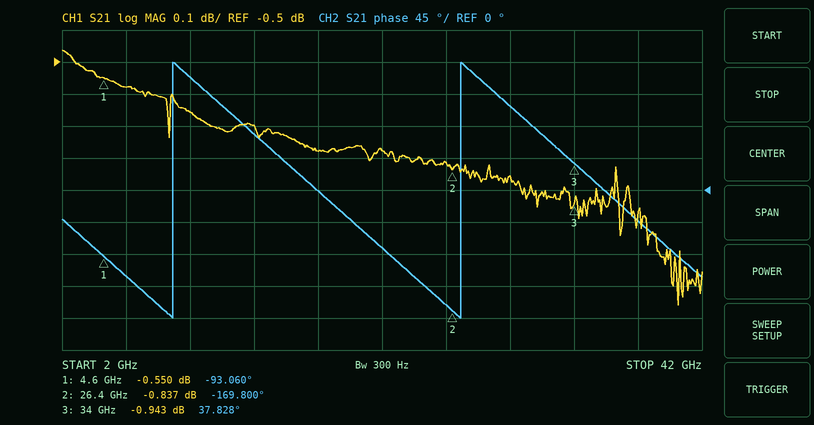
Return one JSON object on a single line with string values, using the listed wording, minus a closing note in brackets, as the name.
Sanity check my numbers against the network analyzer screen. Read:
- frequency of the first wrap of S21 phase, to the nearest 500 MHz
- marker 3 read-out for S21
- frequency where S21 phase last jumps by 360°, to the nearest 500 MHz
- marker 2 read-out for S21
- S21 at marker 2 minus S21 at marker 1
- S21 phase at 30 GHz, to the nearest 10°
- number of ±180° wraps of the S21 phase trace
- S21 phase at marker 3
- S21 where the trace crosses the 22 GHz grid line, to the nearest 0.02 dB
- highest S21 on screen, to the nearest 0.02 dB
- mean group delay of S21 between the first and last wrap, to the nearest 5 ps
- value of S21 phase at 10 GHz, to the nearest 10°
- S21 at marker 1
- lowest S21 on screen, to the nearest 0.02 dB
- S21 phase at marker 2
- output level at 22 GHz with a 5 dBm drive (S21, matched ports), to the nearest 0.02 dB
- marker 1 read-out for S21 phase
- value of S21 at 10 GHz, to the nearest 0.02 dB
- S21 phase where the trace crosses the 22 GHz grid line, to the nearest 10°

{"frequency of the first wrap of S21 phase, to the nearest 500 MHz": "9.0 GHz", "marker 3 read-out for S21": "-0.943 dB", "frequency where S21 phase last jumps by 360°, to the nearest 500 MHz": "27.0 GHz", "marker 2 read-out for S21": "-0.837 dB", "S21 at marker 2 minus S21 at marker 1": "-0.287 dB", "S21 phase at 30 GHz, to the nearest 10°": "120°", "number of ±180° wraps of the S21 phase trace": "2", "S21 phase at marker 3": "37.828°", "S21 where the trace crosses the 22 GHz grid line, to the nearest 0.02 dB": "-0.78 dB", "highest S21 on screen, to the nearest 0.02 dB": "-0.46 dB", "mean group delay of S21 between the first and last wrap, to the nearest 5 ps": "55 ps", "value of S21 phase at 10 GHz, to the nearest 10°": "160°", "S21 at marker 1": "-0.550 dB", "lowest S21 on screen, to the nearest 0.02 dB": "-1.26 dB", "S21 phase at marker 2": "-169.800°", "output level at 22 GHz with a 5 dBm drive (S21, matched ports), to the nearest 0.02 dB": "4.22 dBm", "marker 1 read-out for S21 phase": "-93.060°", "value of S21 at 10 GHz, to the nearest 0.02 dB": "-0.66 dB", "S21 phase where the trace crosses the 22 GHz grid line, to the nearest 10°": "-80°"}
